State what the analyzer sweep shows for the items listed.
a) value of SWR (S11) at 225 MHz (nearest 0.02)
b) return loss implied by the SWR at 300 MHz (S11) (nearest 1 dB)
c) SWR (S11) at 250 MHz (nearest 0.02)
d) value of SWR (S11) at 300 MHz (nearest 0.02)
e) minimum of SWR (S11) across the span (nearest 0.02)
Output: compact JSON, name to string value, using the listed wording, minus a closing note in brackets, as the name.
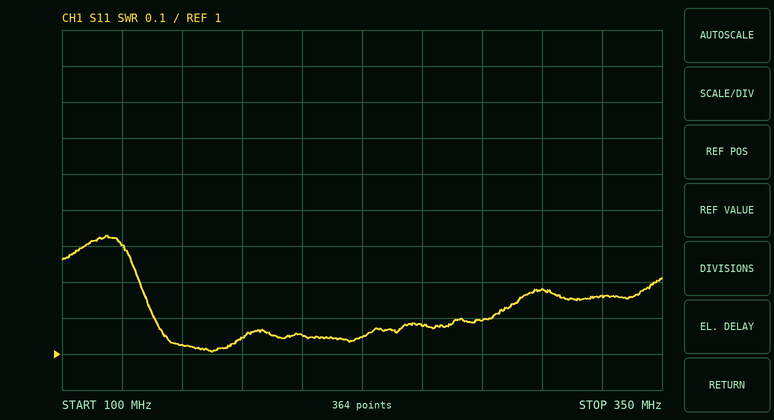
{"value of SWR (S11) at 225 MHz": "1.04", "return loss implied by the SWR at 300 MHz (S11)": "22 dB", "SWR (S11) at 250 MHz": "1.08", "value of SWR (S11) at 300 MHz": "1.18", "minimum of SWR (S11) across the span": "1.00"}
